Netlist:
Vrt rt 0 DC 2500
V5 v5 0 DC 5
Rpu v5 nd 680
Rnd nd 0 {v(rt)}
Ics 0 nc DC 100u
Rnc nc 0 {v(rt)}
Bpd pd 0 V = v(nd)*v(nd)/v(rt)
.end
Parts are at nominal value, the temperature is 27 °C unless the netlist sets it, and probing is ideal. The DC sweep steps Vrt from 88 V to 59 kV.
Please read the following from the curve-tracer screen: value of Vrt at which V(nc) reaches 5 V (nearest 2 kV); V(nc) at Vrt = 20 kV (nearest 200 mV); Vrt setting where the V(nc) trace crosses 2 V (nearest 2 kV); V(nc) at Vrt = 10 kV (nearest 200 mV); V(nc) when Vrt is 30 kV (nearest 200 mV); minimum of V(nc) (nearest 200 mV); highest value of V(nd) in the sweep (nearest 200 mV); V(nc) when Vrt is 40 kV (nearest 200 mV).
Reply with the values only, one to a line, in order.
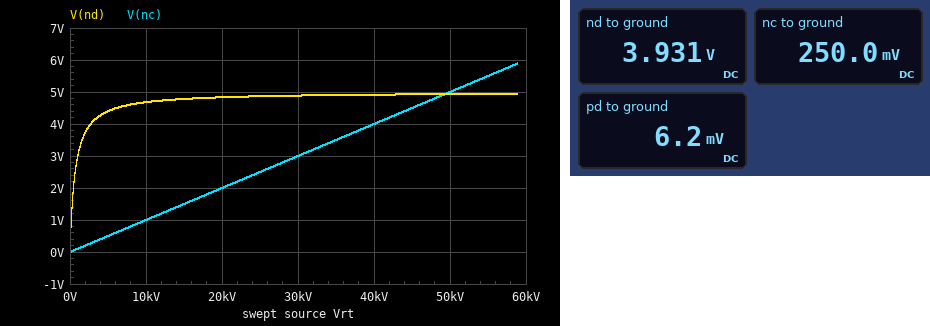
50 kV
2.0 V
20 kV
1.0 V
3.0 V
0 V
5.0 V
4.0 V
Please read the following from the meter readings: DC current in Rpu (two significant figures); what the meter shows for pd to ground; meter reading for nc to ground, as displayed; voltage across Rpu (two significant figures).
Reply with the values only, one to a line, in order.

1.6 mA
6.2 mV
250.0 mV
1.1 V
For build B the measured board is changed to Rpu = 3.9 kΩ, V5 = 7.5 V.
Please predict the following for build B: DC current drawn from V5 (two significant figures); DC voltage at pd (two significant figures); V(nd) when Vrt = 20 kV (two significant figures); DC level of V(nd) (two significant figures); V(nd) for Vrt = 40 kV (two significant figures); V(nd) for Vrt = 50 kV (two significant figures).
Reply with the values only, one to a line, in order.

1.2 mA
3.4 mV
6.3 V
2.9 V
6.8 V
7.0 V
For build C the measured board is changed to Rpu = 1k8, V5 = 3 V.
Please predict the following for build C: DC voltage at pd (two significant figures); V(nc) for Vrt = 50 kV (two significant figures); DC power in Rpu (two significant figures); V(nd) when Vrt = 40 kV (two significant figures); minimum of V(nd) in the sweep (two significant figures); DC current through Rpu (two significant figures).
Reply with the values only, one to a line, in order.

1.2 mV
5.0 V
880 µW
2.9 V
140 mV
700 µA
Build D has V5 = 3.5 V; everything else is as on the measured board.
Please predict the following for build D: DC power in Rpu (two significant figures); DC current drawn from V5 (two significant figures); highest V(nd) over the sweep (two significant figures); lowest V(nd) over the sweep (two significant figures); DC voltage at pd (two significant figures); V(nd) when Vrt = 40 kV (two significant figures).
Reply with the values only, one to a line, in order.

820 µW
1.1 mA
3.5 V
400 mV
3.0 mV
3.4 V
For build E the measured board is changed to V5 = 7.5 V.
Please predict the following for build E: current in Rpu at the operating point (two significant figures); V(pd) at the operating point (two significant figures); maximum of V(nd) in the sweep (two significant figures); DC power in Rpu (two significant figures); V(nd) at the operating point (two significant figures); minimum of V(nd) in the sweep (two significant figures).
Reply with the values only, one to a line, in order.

2.4 mA
14 mV
7.4 V
3.8 mW
5.9 V
860 mV
